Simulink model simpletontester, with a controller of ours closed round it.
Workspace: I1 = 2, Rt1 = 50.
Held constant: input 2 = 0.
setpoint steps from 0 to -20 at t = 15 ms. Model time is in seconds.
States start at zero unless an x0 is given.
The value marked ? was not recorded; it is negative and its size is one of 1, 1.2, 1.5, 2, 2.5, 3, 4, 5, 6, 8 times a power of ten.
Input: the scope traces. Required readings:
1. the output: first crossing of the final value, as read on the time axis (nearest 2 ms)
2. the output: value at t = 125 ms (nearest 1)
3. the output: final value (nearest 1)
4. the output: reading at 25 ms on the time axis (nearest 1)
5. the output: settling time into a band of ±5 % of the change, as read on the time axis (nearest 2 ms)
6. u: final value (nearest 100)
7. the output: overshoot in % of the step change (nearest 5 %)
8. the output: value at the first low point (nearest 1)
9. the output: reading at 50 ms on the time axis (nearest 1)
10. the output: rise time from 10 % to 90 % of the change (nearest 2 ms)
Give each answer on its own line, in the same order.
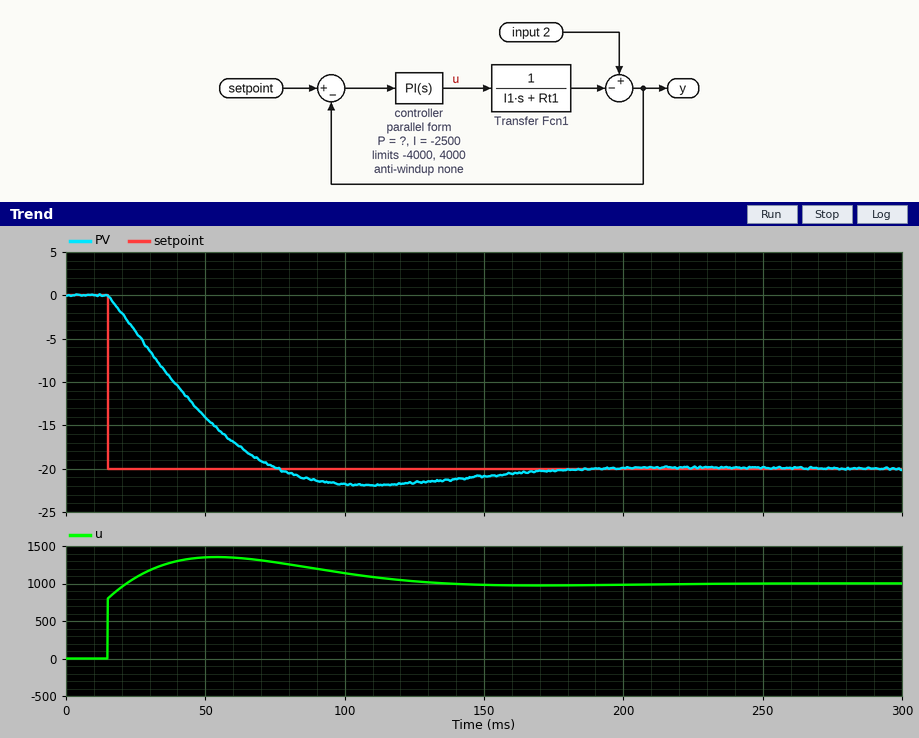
76 ms
-22
-20
-4
146 ms
1000
10 %
-22
-14
44 ms
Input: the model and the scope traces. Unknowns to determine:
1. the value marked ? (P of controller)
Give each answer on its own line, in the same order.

-40
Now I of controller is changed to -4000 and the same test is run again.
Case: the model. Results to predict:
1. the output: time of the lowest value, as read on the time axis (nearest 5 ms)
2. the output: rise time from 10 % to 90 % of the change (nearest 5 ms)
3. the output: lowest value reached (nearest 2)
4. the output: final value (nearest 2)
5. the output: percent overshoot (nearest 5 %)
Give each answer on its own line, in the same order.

85 ms
30 ms
-24
-20
20 %
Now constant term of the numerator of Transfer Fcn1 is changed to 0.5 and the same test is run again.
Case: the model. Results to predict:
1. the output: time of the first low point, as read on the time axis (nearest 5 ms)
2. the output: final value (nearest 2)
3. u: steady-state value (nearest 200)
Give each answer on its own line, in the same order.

170 ms
-20
2000
